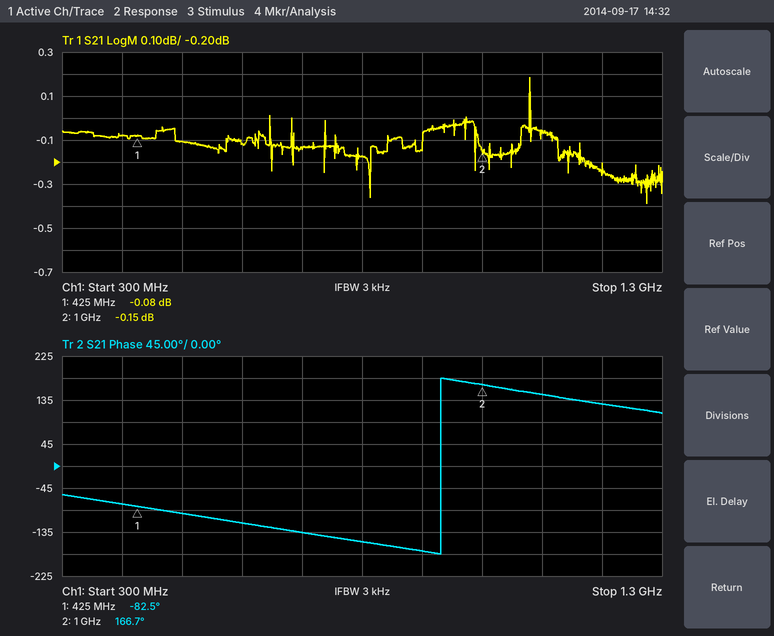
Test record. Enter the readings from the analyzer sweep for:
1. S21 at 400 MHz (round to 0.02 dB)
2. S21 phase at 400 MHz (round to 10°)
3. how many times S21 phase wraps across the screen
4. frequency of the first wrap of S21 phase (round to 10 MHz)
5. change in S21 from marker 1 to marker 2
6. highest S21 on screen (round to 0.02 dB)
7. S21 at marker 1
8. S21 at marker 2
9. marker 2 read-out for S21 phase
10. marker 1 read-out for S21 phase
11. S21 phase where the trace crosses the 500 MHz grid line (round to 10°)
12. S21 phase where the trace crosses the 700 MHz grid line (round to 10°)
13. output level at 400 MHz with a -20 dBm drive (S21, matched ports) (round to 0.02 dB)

-0.08 dB
-80°
1
930 MHz
-0.07 dB
0.18 dB
-0.08 dB
-0.15 dB
166.7°
-82.5°
-100°
-140°
-20.08 dBm
